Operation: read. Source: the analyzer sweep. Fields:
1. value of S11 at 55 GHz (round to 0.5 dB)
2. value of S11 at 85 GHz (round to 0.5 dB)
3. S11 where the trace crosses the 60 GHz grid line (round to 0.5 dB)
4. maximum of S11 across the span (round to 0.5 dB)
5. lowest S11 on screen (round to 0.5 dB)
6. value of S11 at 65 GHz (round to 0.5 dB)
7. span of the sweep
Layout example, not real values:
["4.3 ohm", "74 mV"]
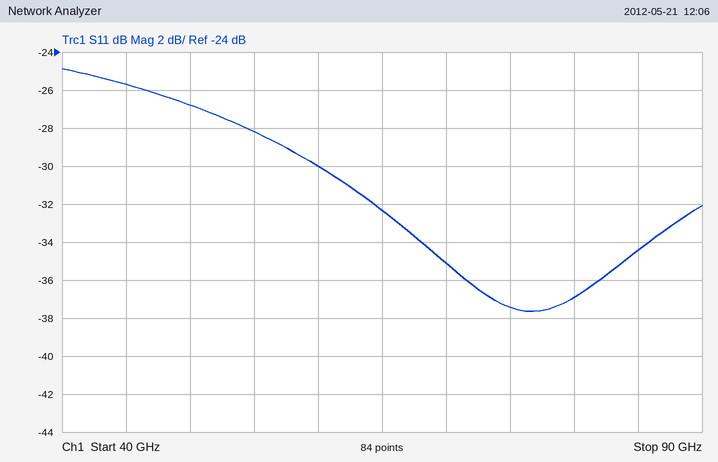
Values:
["-28.0 dB", "-34.5 dB", "-30.0 dB", "-25.0 dB", "-37.5 dB", "-32.5 dB", "50 GHz"]
